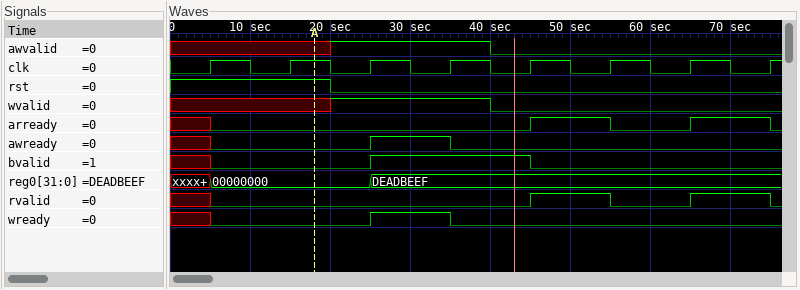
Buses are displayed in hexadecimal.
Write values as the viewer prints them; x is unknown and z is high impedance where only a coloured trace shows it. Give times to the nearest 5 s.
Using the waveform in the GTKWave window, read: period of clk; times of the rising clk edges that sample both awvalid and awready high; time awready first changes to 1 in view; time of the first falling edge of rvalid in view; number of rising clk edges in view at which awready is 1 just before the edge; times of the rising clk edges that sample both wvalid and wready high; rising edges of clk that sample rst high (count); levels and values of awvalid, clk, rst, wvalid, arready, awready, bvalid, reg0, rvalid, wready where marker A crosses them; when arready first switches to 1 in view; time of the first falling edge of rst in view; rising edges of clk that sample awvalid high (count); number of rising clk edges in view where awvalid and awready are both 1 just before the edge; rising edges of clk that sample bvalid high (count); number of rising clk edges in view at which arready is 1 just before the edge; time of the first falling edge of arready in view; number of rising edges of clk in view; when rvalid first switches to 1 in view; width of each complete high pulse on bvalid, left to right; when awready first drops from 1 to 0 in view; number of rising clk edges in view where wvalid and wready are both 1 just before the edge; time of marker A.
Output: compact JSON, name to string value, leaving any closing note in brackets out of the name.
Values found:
{"period of clk": "10 s", "times of the rising clk edges that sample both awvalid and awready high": "35 s", "time awready first changes to 1 in view": "25 s", "time of the first falling edge of rvalid in view": "55 s", "number of rising clk edges in view at which awready is 1 just before the edge": "1", "times of the rising clk edges that sample both wvalid and wready high": "35 s", "rising edges of clk that sample rst high": "2", "levels and values of awvalid, clk, rst, wvalid, arready, awready, bvalid, reg0, rvalid, wready where marker A crosses them": "awvalid=x, clk=1, rst=1, wvalid=x, arready=0, awready=0, bvalid=0, reg0=00000000, rvalid=0, wready=0", "when arready first switches to 1 in view": "45 s", "time of the first falling edge of rst in view": "20 s", "rising edges of clk that sample awvalid high": "2", "number of rising clk edges in view where awvalid and awready are both 1 just before the edge": "1", "rising edges of clk that sample bvalid high": "2", "number of rising clk edges in view at which arready is 1 just before the edge": "2", "time of the first falling edge of arready in view": "55 s", "number of rising edges of clk in view": "8", "when rvalid first switches to 1 in view": "45 s", "width of each complete high pulse on bvalid, left to right": "20 s", "when awready first drops from 1 to 0 in view": "35 s", "number of rising clk edges in view where wvalid and wready are both 1 just before the edge": "1", "time of marker A": "20 s"}
